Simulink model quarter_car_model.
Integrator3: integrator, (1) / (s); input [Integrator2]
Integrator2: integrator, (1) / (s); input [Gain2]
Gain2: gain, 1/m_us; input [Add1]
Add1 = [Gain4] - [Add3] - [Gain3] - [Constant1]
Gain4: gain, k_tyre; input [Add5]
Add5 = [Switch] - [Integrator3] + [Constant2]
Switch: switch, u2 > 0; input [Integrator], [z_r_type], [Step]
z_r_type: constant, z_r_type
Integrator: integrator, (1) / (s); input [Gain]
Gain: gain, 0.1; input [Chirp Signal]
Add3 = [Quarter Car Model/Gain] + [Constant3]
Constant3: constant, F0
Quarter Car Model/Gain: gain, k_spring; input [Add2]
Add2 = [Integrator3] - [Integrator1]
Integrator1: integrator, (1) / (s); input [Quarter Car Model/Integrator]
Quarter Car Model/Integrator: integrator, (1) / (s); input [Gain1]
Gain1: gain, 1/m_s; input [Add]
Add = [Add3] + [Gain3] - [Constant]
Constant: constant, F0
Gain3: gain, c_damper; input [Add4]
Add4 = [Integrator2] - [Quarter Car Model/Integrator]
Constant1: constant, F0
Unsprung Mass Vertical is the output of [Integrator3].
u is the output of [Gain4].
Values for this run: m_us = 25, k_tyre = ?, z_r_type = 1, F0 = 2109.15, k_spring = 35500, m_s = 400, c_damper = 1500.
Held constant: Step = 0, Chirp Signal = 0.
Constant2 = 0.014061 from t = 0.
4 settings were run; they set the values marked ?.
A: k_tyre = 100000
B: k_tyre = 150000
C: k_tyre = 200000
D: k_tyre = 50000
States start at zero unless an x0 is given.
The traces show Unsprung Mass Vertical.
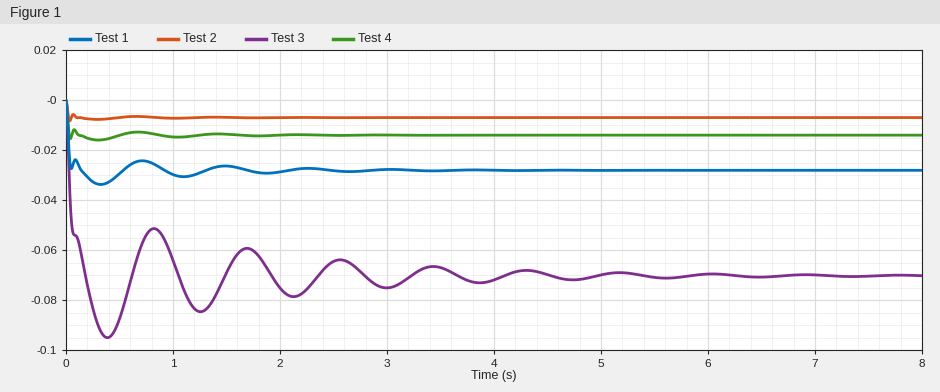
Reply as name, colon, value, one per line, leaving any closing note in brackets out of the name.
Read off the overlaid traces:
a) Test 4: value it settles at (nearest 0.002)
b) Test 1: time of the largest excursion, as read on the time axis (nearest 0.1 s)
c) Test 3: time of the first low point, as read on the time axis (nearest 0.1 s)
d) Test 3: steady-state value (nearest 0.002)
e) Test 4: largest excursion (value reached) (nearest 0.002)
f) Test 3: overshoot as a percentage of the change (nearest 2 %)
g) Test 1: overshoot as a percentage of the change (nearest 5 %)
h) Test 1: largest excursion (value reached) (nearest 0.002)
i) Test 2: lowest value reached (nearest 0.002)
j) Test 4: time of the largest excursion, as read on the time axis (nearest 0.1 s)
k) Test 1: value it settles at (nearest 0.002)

Test 4: value it settles at: -0.014
Test 1: time of the largest excursion, as read on the time axis: 0.3 s
Test 3: time of the first low point, as read on the time axis: 0.4 s
Test 3: steady-state value: -0.070
Test 4: largest excursion (value reached): -0.016
Test 3: overshoot as a percentage of the change: 36 %
Test 1: overshoot as a percentage of the change: 20 %
Test 1: largest excursion (value reached): -0.034
Test 2: lowest value reached: -0.008
Test 4: time of the largest excursion, as read on the time axis: 0.3 s
Test 1: value it settles at: -0.028
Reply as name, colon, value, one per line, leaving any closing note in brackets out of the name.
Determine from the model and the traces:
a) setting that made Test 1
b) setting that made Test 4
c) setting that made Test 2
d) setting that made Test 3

setting that made Test 1: A
setting that made Test 4: B
setting that made Test 2: C
setting that made Test 3: D
